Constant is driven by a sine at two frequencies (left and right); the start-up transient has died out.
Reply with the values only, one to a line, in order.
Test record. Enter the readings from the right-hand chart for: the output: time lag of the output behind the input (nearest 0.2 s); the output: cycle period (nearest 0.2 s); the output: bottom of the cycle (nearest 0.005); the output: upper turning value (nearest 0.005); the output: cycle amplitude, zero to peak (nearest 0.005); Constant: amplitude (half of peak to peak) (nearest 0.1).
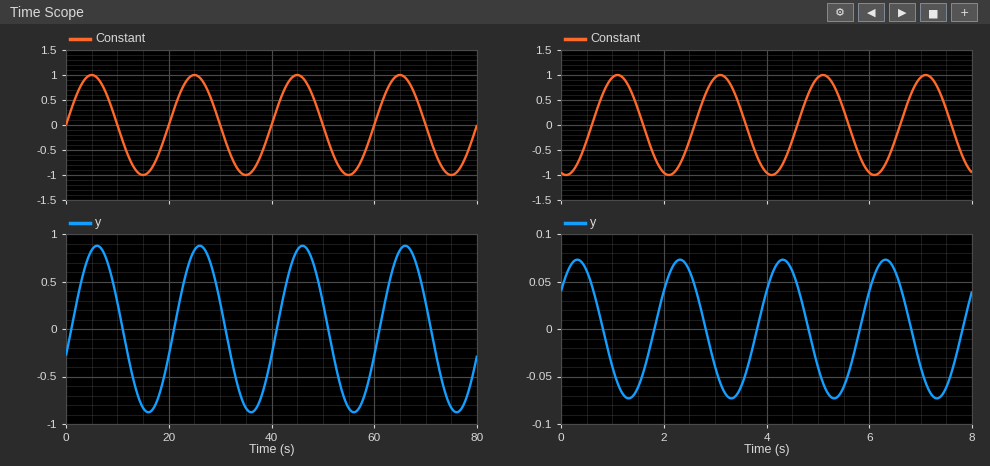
1.2 s
2.0 s
-0.075
0.075
0.075
1.0
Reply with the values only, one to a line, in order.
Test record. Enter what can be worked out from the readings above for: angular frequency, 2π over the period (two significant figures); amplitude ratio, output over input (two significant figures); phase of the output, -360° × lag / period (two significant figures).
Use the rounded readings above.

3.1 rad/s
0.075
-220°
